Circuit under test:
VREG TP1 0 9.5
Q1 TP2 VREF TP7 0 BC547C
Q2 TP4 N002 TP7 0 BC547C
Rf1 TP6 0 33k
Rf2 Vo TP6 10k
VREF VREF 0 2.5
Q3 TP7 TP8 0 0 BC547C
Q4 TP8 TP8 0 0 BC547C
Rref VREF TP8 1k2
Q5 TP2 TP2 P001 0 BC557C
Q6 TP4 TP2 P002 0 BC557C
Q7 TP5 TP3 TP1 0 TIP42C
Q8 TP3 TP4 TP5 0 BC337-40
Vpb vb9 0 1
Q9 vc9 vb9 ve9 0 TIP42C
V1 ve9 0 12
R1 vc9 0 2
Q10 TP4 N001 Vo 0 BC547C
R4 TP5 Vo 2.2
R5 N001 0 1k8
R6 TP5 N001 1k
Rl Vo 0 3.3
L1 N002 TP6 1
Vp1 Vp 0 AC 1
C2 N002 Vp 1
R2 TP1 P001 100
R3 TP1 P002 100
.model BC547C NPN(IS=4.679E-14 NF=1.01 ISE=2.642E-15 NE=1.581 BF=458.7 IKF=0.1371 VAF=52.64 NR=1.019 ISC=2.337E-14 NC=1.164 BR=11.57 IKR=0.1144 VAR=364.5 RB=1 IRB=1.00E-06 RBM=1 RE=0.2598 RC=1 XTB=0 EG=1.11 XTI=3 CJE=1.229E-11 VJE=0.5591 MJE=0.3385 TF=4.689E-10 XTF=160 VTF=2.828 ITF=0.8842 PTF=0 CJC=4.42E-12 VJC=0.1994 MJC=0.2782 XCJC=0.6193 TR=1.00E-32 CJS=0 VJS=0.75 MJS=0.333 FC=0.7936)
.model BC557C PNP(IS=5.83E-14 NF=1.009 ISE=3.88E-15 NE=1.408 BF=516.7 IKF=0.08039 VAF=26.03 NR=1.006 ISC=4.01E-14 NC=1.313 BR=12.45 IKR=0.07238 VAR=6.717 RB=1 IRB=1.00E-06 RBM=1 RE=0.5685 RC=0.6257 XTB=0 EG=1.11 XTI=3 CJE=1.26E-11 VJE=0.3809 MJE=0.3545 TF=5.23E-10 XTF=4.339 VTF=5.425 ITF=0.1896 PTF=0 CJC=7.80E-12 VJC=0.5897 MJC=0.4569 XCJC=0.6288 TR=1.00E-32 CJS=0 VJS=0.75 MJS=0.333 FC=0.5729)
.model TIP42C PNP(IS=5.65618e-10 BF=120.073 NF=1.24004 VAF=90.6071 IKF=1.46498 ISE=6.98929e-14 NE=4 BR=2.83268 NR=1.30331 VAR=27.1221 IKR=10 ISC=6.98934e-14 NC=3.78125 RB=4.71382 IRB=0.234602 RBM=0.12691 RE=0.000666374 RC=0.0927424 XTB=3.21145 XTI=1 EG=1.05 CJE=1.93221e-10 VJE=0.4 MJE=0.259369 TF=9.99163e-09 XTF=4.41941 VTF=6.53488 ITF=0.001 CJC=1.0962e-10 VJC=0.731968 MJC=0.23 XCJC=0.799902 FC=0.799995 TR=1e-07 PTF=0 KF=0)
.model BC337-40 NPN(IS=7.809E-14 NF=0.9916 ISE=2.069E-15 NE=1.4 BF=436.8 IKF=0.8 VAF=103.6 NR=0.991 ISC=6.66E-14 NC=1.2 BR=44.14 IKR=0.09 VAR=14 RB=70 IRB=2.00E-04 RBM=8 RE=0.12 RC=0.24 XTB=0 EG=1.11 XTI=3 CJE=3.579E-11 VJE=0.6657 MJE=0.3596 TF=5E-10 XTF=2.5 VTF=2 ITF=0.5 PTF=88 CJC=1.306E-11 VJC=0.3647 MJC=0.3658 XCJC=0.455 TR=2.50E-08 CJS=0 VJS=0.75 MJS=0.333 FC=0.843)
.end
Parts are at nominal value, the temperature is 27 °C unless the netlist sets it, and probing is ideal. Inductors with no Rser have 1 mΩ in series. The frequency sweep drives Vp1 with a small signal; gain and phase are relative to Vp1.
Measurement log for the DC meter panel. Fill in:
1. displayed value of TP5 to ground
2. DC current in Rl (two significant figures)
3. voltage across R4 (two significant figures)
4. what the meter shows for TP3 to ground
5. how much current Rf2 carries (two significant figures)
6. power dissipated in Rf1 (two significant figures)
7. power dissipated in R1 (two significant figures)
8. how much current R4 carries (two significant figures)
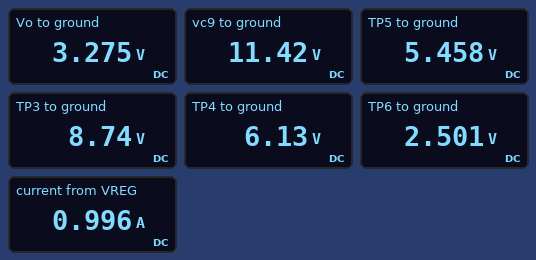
5.458 V
990 mA
2.2 V
8.74 V
77 µA
190 µW
65 W
990 mA
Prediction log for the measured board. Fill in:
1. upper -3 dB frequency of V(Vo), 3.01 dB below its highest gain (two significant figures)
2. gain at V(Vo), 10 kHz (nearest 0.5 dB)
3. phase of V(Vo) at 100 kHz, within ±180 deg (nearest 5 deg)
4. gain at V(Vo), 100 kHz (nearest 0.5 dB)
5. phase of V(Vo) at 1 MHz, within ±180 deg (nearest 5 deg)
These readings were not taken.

120 kHz
55.0 dB
135 deg
53.0 dB
55 deg
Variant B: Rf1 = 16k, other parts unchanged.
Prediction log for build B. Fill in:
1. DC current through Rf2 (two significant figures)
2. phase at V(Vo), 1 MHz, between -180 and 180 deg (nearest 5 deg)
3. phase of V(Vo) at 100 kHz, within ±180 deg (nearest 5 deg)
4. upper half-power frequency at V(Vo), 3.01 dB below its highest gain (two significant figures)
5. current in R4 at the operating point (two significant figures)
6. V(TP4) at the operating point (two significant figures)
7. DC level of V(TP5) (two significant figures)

160 µA
60 deg
130 deg
100 kHz
1.2 A
7.5 V
6.8 V
